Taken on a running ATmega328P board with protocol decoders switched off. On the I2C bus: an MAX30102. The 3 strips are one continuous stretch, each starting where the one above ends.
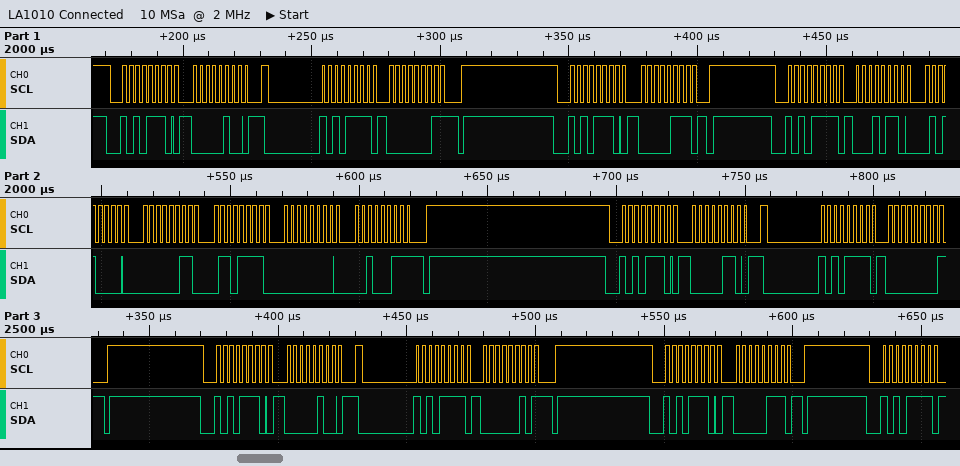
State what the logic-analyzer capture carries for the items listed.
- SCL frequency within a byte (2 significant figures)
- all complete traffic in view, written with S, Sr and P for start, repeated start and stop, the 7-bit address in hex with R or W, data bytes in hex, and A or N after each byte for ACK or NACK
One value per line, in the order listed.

400 kHz
S 57W A 04 A Sr 57R A 01 N P S 57W A 07 A P S 57R A 16 A 50 A 03 A 6F A 00 A 23 N P S 57W A 06 A Sr 57R A 00 N P S 57W A 04 A Sr 57R A 02 N P S 57W A 07 A P S 57R A
